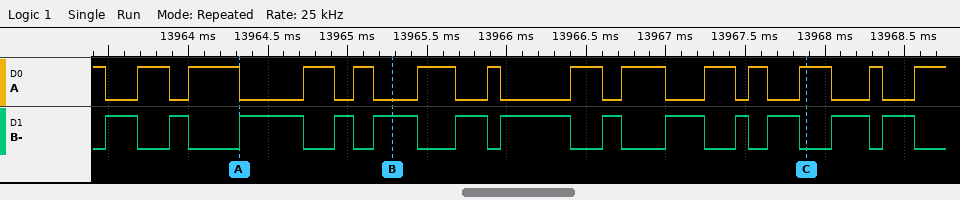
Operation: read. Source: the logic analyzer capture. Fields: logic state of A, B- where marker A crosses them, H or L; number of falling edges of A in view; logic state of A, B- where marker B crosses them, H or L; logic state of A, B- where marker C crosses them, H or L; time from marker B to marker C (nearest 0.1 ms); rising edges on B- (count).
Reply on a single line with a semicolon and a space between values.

A=L, B-=H; 13; A=L, B-=H; A=H, B-=L; 2.6 ms; 13
